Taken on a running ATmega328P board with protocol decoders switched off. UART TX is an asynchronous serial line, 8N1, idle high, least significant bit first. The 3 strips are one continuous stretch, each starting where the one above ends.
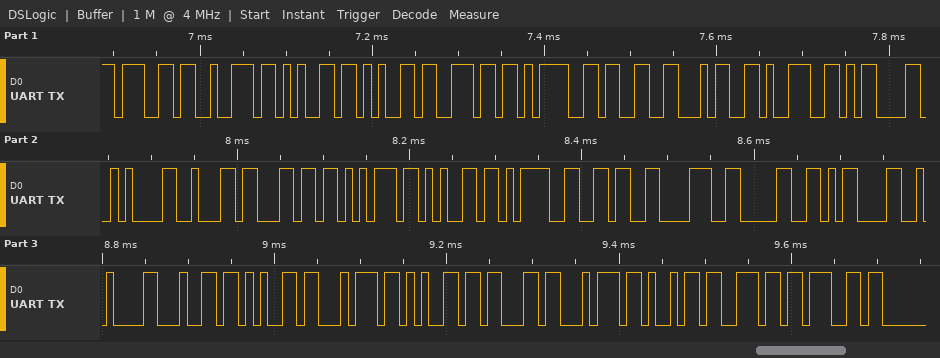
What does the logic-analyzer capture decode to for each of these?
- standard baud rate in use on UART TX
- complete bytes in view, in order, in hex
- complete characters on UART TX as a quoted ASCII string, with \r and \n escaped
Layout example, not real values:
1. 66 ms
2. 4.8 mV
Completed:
1. 115200 baud
2. 67 72 65 65 6E 3D 33 34 39 0D 0A 62 6C 75 65 3D 36 38 30 0D 0A 64 65 74 65 63 74 69 6E 67
3. "green=349\r\nblue=680\r\ndetecting"
